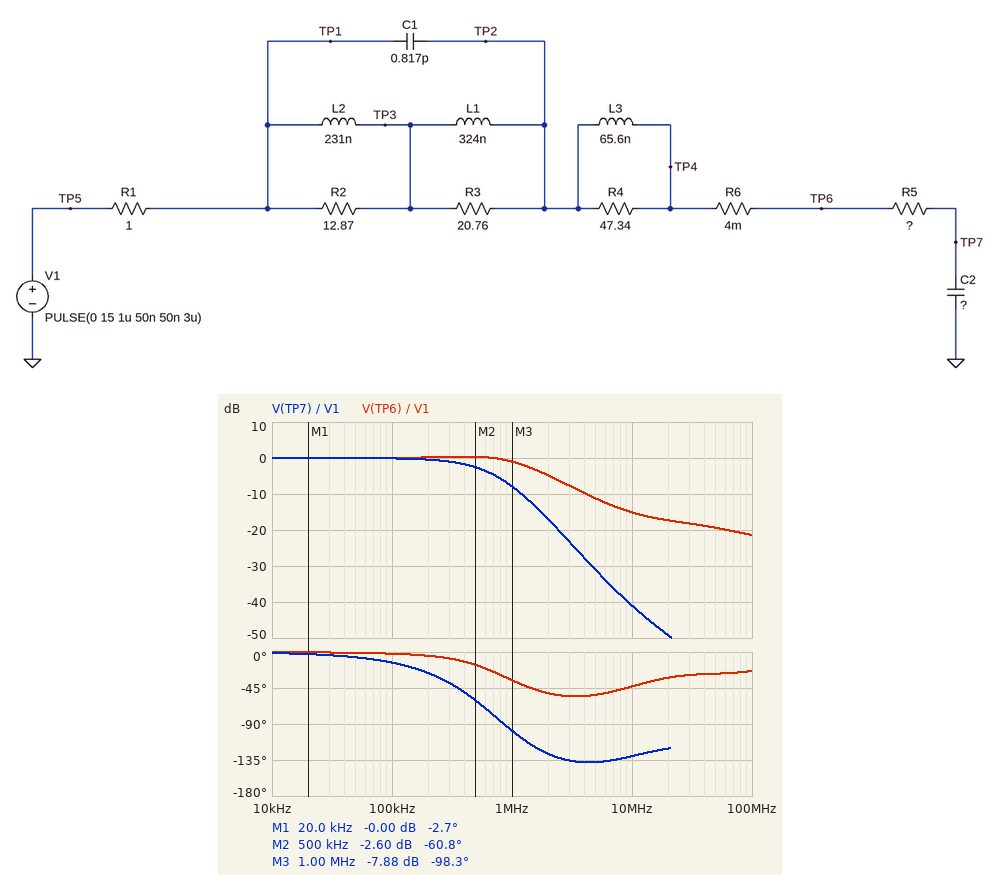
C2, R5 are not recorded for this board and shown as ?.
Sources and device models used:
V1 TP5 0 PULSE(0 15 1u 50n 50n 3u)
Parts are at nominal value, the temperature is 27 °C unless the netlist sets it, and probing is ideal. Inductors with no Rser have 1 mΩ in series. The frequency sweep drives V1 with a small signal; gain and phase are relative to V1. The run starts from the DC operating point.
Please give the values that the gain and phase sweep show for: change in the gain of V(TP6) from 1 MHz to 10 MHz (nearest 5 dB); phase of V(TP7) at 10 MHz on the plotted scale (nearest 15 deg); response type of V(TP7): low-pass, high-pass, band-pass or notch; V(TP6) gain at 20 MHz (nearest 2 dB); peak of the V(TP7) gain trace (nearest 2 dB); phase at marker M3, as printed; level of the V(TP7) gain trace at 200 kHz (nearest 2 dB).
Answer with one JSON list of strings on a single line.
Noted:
["-15 dB", "-135 deg", "low-pass", "-18 dB", "0 dB", "-98.3 deg", "0 dB"]
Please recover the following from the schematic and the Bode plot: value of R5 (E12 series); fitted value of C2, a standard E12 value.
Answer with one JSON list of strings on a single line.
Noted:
["5.6 Ω", "56 nF"]
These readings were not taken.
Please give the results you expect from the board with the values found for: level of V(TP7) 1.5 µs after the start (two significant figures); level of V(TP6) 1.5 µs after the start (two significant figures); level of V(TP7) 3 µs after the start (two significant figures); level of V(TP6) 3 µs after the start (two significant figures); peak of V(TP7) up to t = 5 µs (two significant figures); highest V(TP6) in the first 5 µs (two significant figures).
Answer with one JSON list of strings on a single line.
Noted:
["11 V", "16 V", "15 V", "15 V", "15 V", "16 V"]
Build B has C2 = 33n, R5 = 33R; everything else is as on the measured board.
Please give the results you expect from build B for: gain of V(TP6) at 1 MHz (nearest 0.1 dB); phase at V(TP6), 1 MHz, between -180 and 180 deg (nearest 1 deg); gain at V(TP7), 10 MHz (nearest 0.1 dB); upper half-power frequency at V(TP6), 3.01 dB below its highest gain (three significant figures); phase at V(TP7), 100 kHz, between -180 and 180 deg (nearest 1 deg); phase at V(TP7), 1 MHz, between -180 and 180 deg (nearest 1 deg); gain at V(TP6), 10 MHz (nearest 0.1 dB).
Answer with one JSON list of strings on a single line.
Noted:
["-0.3 dB", "-7 deg", "-41.2 dB", "6.02 MHz", "-35 deg", "-88 deg", "-4.5 dB"]
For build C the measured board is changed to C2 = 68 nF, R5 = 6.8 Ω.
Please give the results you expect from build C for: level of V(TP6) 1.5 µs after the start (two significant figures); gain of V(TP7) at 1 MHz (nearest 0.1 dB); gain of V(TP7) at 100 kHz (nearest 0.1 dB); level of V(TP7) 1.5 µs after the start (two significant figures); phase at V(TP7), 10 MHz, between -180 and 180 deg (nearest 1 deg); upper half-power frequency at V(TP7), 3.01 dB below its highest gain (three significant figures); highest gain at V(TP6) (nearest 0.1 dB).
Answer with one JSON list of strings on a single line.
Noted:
["15 V", "-11.0 dB", "-0.3 dB", "8.5 V", "-129 deg", "348 kHz", "0.1 dB"]
